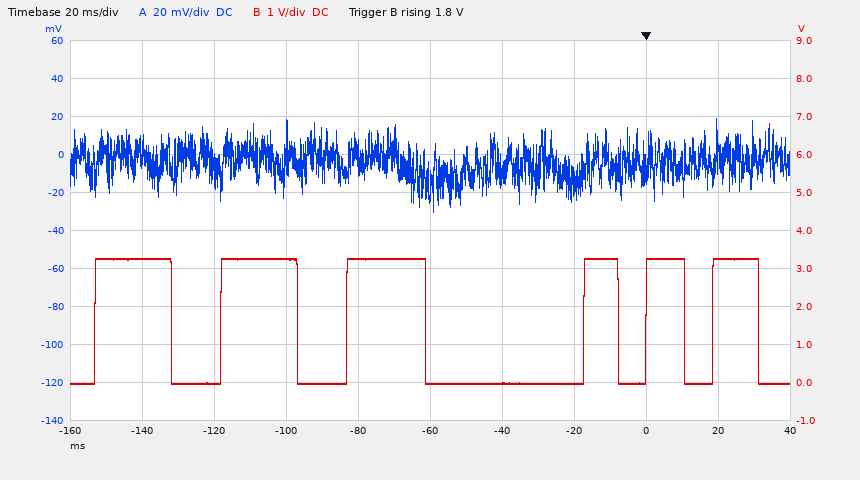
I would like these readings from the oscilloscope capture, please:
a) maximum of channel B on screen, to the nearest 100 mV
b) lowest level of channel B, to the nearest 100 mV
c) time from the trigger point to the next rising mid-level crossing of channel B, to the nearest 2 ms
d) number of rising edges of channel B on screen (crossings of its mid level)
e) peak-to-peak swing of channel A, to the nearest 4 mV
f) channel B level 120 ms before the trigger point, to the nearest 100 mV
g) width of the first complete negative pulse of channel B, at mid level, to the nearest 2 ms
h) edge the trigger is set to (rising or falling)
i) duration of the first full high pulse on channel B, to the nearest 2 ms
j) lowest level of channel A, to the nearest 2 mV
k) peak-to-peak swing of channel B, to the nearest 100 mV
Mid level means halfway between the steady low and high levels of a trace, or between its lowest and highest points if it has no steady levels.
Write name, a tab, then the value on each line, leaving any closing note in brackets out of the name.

maximum of channel B on screen, to the nearest 100 mV	3.3 V
lowest level of channel B, to the nearest 100 mV	0.0 V
time from the trigger point to the next rising mid-level crossing of channel B, to the nearest 2 ms	18 ms
number of rising edges of channel B on screen	6
peak-to-peak swing of channel A, to the nearest 4 mV	48 mV
channel B level 120 ms before the trigger point, to the nearest 100 mV	0.0 V
width of the first complete negative pulse of channel B, at mid level, to the nearest 2 ms	14 ms
edge the trigger is set to	rising
duration of the first full high pulse on channel B, to the nearest 2 ms	22 ms
lowest level of channel A, to the nearest 2 mV	-30 mV
peak-to-peak swing of channel B, to the nearest 100 mV	3.3 V
